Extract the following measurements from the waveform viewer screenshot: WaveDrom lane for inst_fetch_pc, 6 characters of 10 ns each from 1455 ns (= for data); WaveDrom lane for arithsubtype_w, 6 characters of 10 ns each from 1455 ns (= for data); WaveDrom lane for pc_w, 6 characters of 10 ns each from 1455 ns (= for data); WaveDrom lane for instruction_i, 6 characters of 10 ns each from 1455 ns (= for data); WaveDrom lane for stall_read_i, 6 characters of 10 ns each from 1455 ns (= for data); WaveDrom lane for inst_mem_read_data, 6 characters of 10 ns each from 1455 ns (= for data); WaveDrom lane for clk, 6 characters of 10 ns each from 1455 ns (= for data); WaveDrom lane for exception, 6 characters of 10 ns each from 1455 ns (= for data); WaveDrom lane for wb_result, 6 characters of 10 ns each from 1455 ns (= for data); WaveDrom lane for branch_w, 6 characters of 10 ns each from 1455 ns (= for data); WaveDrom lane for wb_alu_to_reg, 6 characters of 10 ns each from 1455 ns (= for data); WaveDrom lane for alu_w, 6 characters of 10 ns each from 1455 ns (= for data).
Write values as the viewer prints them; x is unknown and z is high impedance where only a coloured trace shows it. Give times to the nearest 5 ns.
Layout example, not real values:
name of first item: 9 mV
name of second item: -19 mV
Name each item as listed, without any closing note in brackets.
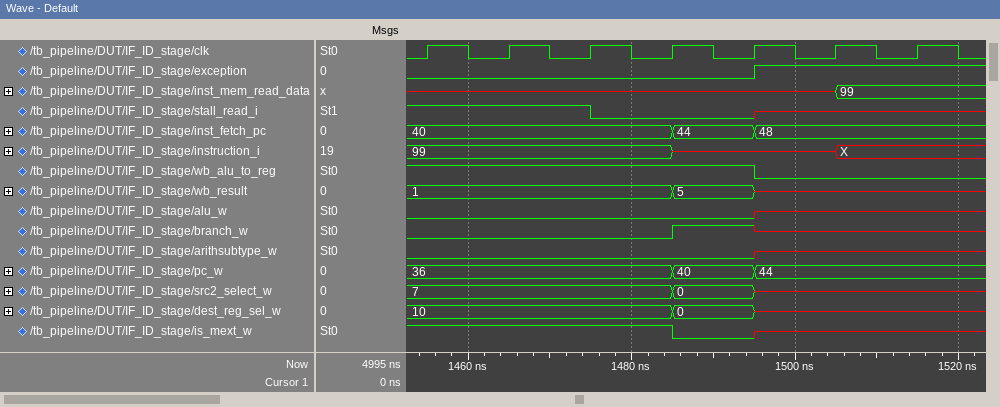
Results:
WaveDrom lane for inst_fetch_pc, 6 characters of 10 ns each from 1455 ns: {name: 'inst_fetch_pc', wave: '=..==.', data: '40 44 48'}
WaveDrom lane for arithsubtype_w, 6 characters of 10 ns each from 1455 ns: {name: 'arithsubtype_w', wave: '0...x.'}
WaveDrom lane for pc_w, 6 characters of 10 ns each from 1455 ns: {name: 'pc_w', wave: '=..==.', data: '36 40 44'}
WaveDrom lane for instruction_i, 6 characters of 10 ns each from 1455 ns: {name: 'instruction_i', wave: '=..x.=', data: '99 X'}
WaveDrom lane for stall_read_i, 6 characters of 10 ns each from 1455 ns: {name: 'stall_read_i', wave: '1.0.x.'}
WaveDrom lane for inst_mem_read_data, 6 characters of 10 ns each from 1455 ns: {name: 'inst_mem_read_data', wave: 'x....=', data: '99'}
WaveDrom lane for clk, 6 characters of 10 ns each from 1455 ns: {name: 'clk', wave: 'p.....'}
WaveDrom lane for exception, 6 characters of 10 ns each from 1455 ns: {name: 'exception', wave: '0...1.'}
WaveDrom lane for wb_result, 6 characters of 10 ns each from 1455 ns: {name: 'wb_result', wave: '=..=x.', data: '1 5'}
WaveDrom lane for branch_w, 6 characters of 10 ns each from 1455 ns: {name: 'branch_w', wave: '0..1x.'}
WaveDrom lane for wb_alu_to_reg, 6 characters of 10 ns each from 1455 ns: {name: 'wb_alu_to_reg', wave: '1...0.'}
WaveDrom lane for alu_w, 6 characters of 10 ns each from 1455 ns: {name: 'alu_w', wave: '0...x.'}
